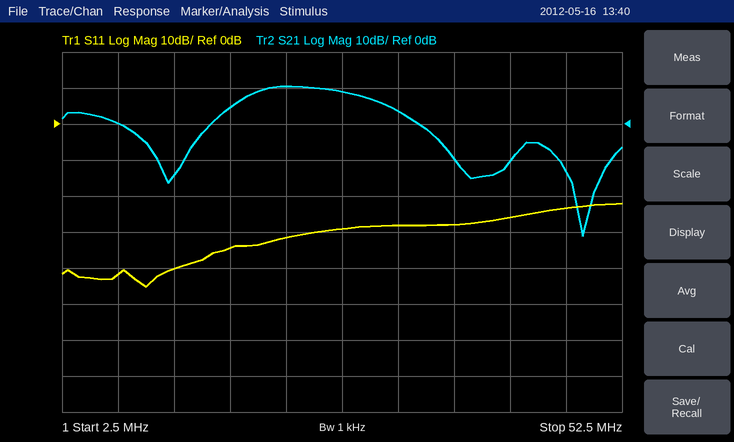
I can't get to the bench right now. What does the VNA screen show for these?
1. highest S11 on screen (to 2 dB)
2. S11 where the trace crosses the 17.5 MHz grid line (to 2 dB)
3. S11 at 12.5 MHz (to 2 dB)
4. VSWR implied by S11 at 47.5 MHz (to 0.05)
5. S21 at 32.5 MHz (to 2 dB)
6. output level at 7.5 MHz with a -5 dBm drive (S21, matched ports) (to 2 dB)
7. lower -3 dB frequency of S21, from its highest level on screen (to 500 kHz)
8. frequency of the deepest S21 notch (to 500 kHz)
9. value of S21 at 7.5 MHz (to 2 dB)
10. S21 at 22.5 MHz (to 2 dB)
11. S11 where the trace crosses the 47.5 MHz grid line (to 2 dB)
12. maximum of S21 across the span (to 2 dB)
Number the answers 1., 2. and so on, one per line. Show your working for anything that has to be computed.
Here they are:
1. -22 dB
2. -34 dB
3. -40 dB
4. |Γ| = 10^(-24/20) = 0.0631; VSWR = (1 + 0.0631)/(1 − 0.0631) ≈ 1.13, so 1.15 to the nearest 0.05
5. 4 dB
6. -5 dBm + (0 dB) = -4 dBm
7. 19.0 MHz
8. 49.0 MHz
9. 0 dB
10. 10 dB
11. -24 dB
12. 10 dB
